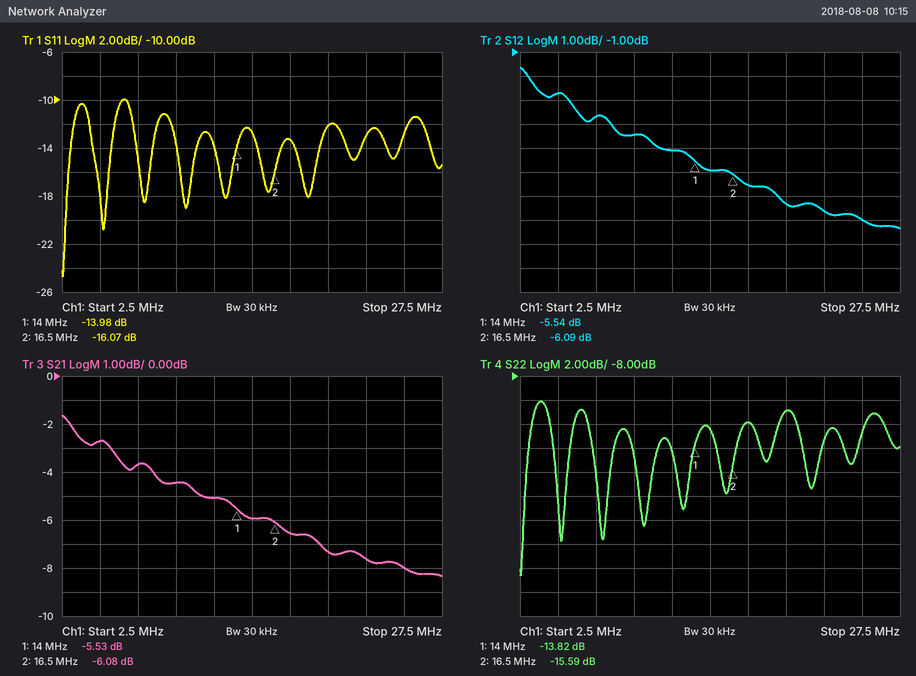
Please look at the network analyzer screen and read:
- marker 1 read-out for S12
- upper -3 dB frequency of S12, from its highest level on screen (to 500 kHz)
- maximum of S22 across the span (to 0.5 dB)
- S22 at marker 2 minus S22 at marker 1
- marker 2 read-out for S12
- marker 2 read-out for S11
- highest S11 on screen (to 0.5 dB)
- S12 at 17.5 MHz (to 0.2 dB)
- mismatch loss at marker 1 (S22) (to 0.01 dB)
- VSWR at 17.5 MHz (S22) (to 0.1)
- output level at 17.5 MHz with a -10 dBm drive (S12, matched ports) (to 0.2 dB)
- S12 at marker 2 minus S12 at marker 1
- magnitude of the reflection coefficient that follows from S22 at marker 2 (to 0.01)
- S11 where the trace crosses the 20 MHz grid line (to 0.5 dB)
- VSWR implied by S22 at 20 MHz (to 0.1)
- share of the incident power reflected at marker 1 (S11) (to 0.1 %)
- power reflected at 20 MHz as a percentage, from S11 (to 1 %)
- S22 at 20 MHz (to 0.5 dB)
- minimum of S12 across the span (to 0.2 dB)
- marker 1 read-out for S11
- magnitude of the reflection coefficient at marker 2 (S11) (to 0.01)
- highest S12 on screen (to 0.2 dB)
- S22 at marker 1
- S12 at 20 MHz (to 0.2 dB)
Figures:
-5.54 dB
11.0 MHz
-10.0 dB
-1.77 dB
-6.09 dB
-16.07 dB
-10.0 dB
-6.6 dB
0.18 dB
1.7
-16.6 dBm
-0.55 dB
0.17
-12.0 dB
1.8
4.0 %
6 %
-11.0 dB
-8.4 dB
-13.98 dB
0.16
-1.6 dB
-13.82 dB
-7.4 dB
